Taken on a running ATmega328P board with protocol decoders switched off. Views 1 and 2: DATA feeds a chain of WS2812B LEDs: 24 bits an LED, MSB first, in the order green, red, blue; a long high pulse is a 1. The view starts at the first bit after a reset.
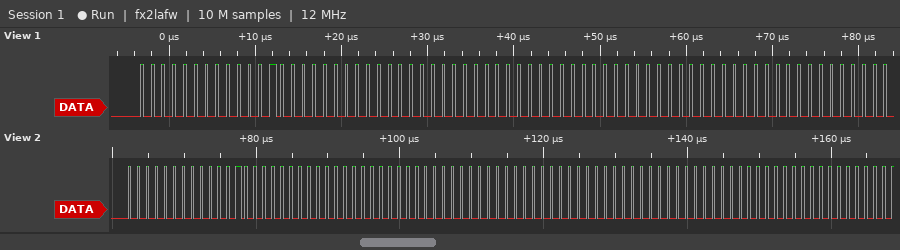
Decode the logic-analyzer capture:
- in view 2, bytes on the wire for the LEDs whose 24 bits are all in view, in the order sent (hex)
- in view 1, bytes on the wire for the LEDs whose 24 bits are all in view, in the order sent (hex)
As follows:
00 08 00 00 00 00 00 00 00
00 08 00 00 00 00
